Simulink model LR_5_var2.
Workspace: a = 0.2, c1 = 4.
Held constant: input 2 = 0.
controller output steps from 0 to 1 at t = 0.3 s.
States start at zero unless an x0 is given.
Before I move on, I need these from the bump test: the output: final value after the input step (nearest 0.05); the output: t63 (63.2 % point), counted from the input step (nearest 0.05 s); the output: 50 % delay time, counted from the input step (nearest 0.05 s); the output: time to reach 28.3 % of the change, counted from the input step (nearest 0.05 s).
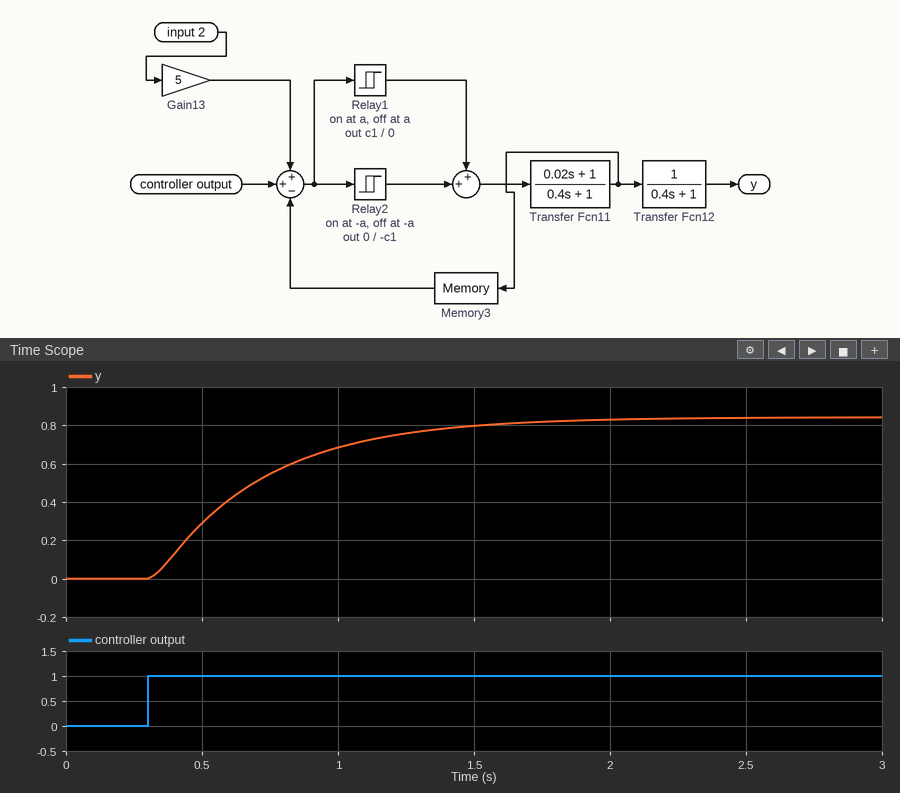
0.85
0.45 s
0.30 s
0.15 s
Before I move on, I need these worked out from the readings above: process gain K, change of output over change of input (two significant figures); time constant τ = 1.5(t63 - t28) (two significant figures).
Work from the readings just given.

0.85
0.45 s
